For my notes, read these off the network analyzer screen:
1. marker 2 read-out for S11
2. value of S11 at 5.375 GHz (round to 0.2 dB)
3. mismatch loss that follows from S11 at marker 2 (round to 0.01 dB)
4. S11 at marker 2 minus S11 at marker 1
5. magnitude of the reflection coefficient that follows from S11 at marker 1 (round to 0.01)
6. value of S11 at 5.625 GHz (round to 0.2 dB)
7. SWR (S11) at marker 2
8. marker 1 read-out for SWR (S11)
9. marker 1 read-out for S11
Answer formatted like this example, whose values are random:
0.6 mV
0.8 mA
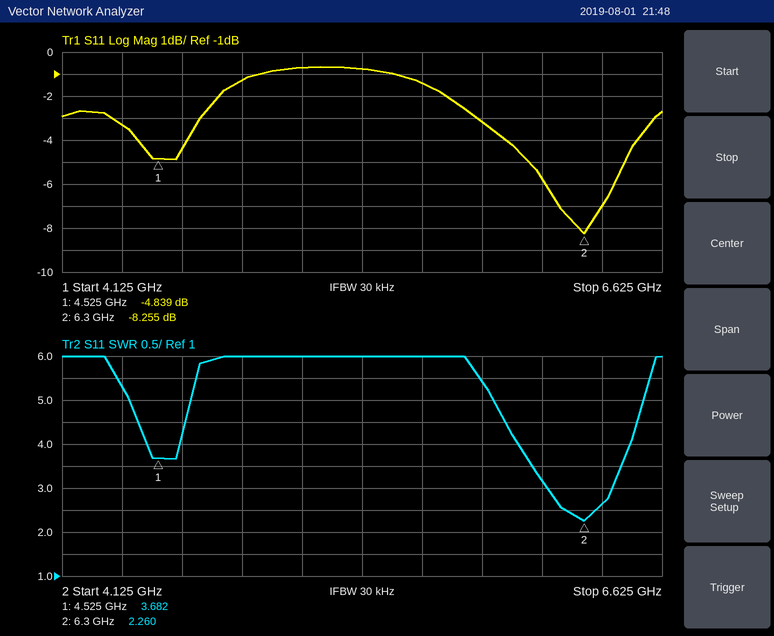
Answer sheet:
-8.255 dB
-0.8 dB
0.70 dB
-3.416 dB
0.57
-1.4 dB
2.260
3.682
-4.839 dB
